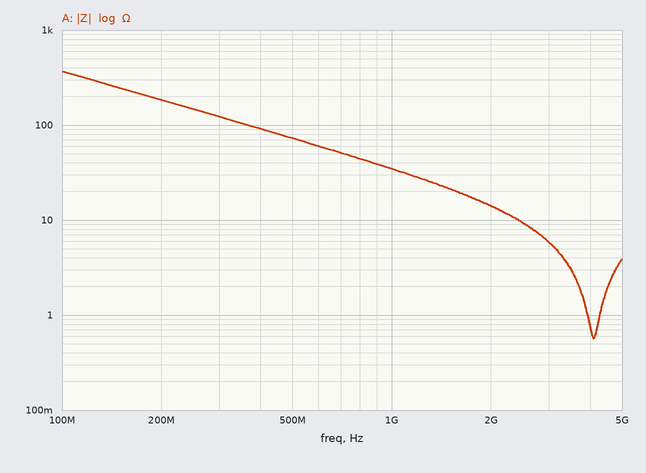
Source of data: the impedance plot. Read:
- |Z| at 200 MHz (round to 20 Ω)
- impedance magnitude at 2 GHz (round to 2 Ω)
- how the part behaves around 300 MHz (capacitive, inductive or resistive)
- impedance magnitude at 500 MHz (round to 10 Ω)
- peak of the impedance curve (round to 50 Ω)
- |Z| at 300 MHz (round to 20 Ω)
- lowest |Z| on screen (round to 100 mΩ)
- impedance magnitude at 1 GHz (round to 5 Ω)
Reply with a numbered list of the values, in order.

1. 180 Ω
2. 14 Ω
3. capacitive
4. 70 Ω
5. 350 Ω
6. 120 Ω
7. 600 mΩ
8. 35 Ω
